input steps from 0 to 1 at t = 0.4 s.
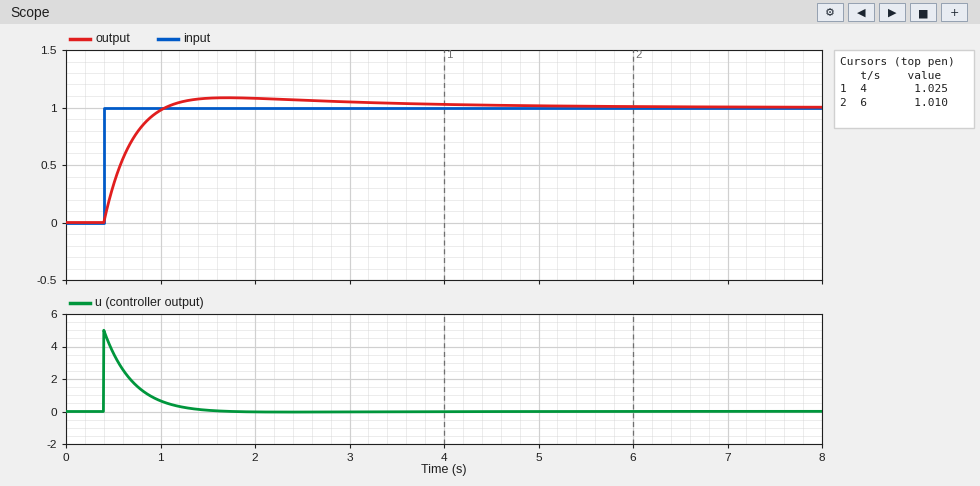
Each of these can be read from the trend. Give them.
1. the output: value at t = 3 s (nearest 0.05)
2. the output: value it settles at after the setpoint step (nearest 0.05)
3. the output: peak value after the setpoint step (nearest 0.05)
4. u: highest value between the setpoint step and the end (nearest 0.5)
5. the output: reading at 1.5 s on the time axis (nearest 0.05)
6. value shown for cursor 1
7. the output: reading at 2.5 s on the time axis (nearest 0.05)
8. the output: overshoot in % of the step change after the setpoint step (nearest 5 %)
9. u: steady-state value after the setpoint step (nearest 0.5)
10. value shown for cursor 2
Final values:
1.05
1.00
1.10
5.0
1.10
1.025
1.05
10 %
0.0
1.010
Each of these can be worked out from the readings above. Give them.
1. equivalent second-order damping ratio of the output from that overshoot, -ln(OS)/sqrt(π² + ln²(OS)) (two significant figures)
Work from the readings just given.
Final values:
0.59
